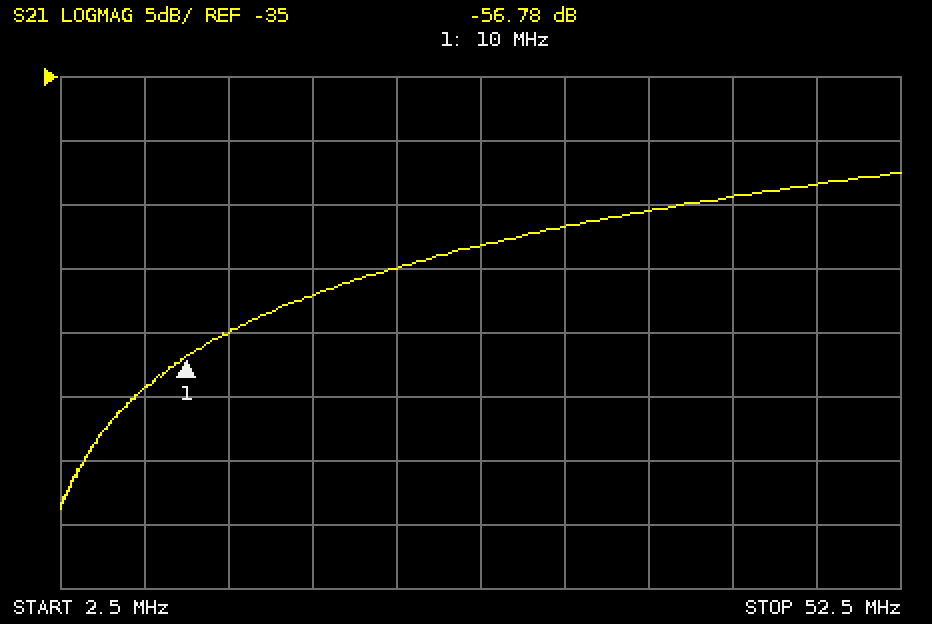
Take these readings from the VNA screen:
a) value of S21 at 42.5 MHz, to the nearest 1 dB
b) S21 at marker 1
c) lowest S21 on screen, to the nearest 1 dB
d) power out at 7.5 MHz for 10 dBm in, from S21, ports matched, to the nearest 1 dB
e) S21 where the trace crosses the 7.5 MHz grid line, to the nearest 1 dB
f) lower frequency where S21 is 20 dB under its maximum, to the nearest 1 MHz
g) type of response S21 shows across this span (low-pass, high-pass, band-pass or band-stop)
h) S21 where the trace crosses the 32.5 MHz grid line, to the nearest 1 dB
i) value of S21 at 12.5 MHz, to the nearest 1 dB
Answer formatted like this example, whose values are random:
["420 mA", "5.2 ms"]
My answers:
["-44 dB", "-56.78 dB", "-69 dB", "-49 dBm", "-59 dB", "5 MHz", "high-pass", "-47 dB", "-55 dB"]
